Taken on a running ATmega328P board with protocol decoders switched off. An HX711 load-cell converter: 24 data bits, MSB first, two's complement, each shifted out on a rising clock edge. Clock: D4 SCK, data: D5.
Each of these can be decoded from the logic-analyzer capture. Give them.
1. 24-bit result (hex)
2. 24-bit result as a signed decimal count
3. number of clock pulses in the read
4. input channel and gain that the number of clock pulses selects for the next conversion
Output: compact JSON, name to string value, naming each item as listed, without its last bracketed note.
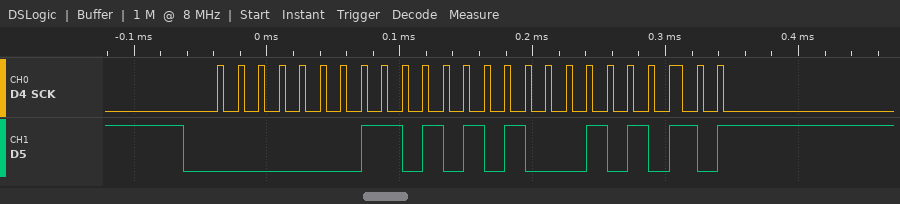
{"24-bit result": "0x01AA2A", "24-bit result as a signed decimal count": "109098", "number of clock pulses in the read": "25", "input channel and gain that the number of clock pulses selects for the next conversion": "channel A, gain 128"}
